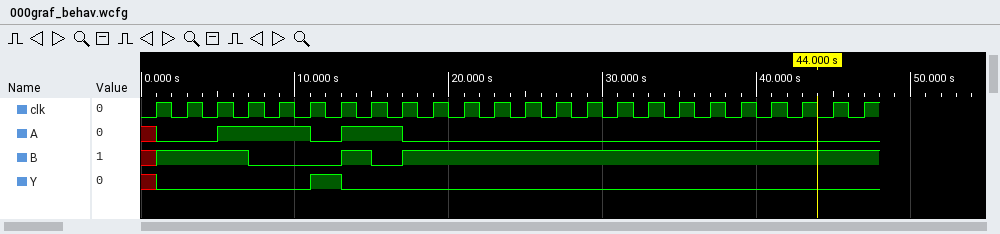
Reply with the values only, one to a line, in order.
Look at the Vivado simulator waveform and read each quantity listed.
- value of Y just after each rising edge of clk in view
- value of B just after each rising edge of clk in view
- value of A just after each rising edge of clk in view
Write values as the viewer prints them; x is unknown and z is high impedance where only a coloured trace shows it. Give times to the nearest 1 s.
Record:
0 0 0 0 0 1 0 0 0 0 0 0 0 0 0 0 0 0 0 0 0 0 0 0
1 1 1 0 0 0 1 0 1 1 1 1 1 1 1 1 1 1 1 1 1 1 1 1
0 0 1 1 1 0 1 1 0 0 0 0 0 0 0 0 0 0 0 0 0 0 0 0
